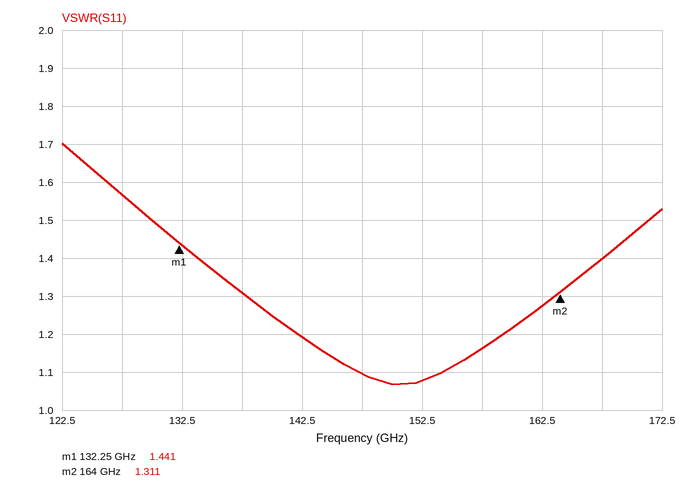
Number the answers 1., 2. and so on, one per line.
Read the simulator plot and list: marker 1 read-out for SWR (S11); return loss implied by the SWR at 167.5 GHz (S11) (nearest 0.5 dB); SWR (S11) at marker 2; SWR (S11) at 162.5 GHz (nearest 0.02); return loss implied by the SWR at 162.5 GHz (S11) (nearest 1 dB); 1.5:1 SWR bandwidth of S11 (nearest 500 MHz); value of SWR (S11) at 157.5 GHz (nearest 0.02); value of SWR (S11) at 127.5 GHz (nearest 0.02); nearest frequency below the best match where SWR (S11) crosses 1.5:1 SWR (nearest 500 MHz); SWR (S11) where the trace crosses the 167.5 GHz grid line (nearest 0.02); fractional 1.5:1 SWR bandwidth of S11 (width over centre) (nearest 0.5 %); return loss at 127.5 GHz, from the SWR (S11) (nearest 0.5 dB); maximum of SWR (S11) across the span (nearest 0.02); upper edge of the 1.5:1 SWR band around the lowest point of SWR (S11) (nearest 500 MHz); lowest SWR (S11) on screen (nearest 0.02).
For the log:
1. 1.441
2. 15.5 dB
3. 1.311
4. 1.28
5. 18 dB
6. 41.5 GHz
7. 1.16
8. 1.56
9. 130.0 GHz
10. 1.40
11. 27.5 %
12. 13.0 dB
13. 1.70
14. 171.5 GHz
15. 1.06
